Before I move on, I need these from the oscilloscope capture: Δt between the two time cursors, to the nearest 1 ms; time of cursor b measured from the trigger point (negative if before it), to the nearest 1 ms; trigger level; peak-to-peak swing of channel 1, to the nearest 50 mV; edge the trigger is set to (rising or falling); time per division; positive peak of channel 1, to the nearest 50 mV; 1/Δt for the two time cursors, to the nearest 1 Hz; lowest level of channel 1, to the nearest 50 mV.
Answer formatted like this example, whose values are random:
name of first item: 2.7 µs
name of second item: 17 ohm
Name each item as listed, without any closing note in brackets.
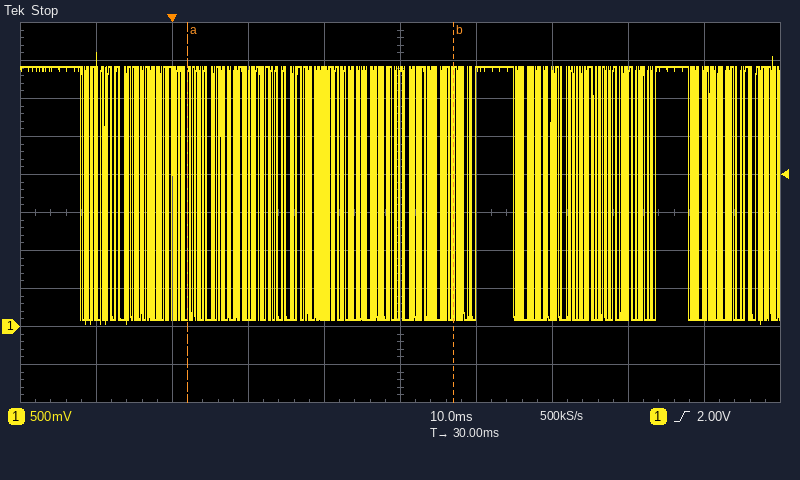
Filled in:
Δt between the two time cursors, to the nearest 1 ms: 35 ms
time of cursor b measured from the trigger point (negative if before it), to the nearest 1 ms: +37 ms
trigger level: 2.00 V
peak-to-peak swing of channel 1, to the nearest 50 mV: 3.55 V
edge the trigger is set to: rising
time per division: 10 ms
positive peak of channel 1, to the nearest 50 mV: 3.60 V
1/Δt for the two time cursors, to the nearest 1 Hz: 29 Hz
lowest level of channel 1, to the nearest 50 mV: 50 mV
